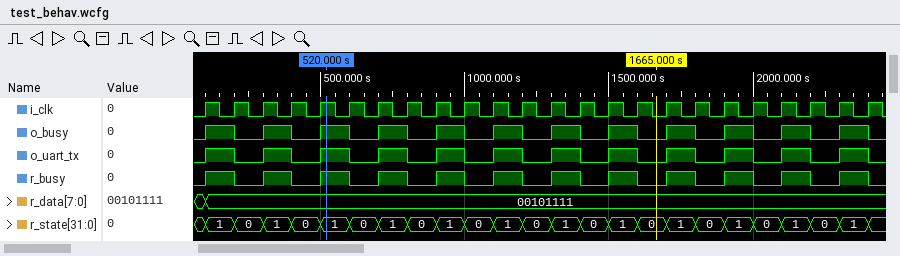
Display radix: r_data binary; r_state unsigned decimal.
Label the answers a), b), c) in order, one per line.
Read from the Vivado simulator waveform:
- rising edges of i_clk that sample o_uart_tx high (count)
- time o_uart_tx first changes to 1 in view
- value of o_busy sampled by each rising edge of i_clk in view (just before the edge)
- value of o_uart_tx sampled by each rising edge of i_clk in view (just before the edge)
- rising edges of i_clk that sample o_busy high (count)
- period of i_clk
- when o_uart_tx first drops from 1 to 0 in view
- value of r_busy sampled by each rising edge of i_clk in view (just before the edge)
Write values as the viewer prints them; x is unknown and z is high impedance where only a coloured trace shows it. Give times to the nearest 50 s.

a) 12
b) 100 s
c) 0 1 0 1 0 1 0 1 0 1 0 1 0 1 0 1 0 1 0 1 0 1 0 1
d) 0 1 0 1 0 1 0 1 0 1 0 1 0 1 0 1 0 1 0 1 0 1 0 1
e) 12
f) 100 s
g) 200 s
h) 0 1 0 1 0 1 0 1 0 1 0 1 0 1 0 1 0 1 0 1 0 1 0 1
